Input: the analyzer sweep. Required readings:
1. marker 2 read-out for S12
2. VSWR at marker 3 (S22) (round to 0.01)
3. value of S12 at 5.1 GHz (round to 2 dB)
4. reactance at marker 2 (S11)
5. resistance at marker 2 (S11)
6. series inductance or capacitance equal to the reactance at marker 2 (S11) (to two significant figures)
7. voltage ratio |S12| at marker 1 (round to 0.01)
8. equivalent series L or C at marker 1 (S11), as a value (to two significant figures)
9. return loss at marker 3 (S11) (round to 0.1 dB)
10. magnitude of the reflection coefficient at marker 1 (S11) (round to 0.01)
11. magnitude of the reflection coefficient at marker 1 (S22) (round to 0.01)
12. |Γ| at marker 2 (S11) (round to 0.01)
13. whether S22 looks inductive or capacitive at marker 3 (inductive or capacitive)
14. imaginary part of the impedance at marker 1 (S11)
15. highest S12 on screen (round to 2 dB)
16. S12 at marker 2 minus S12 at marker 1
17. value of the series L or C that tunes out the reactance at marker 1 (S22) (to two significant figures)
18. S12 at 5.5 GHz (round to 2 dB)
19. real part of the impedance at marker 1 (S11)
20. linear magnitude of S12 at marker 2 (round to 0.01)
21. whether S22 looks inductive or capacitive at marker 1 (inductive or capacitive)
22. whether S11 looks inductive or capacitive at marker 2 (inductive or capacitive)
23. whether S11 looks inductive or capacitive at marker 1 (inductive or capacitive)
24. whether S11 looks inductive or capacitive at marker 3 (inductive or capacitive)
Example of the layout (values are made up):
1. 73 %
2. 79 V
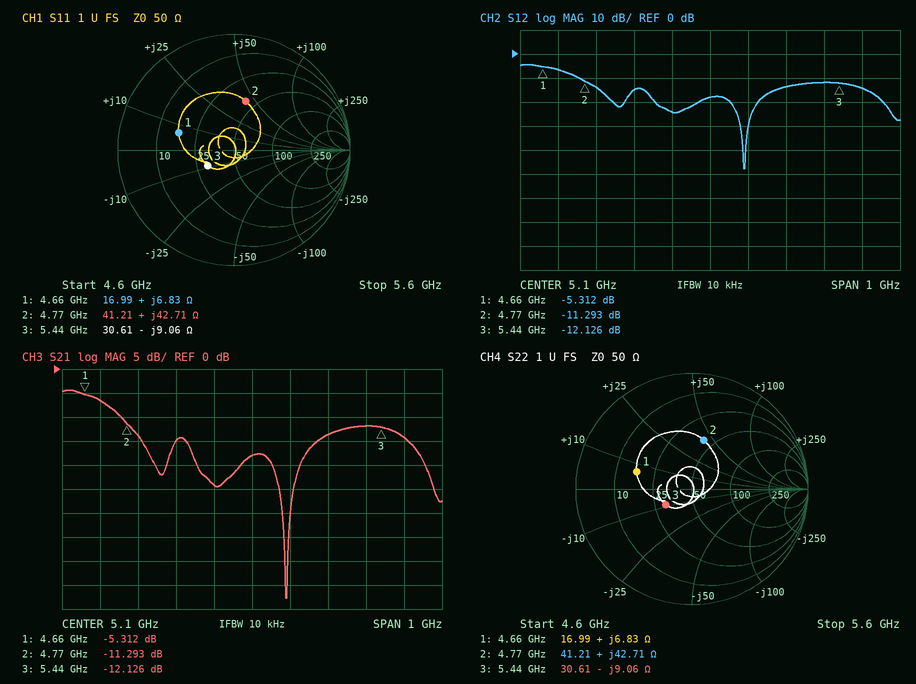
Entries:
1. -11.293 dB
2. 1.72
3. -18 dB
4. +42.71 Ω
5. 41.21 Ω
6. 1.4 nH
7. 0.54
8. 230 pH
9. 11.6 dB
10. 0.50
11. 0.50
12. 0.43
13. capacitive
14. +6.83 Ω
15. -4 dB
16. -5.981 dB
17. 5.0 pF
18. -14 dB
19. 16.99 Ω
20. 0.27
21. inductive
22. inductive
23. inductive
24. capacitive
